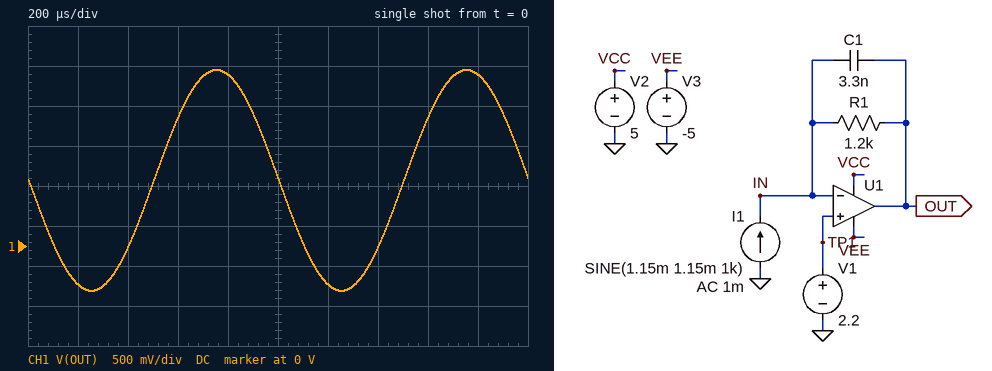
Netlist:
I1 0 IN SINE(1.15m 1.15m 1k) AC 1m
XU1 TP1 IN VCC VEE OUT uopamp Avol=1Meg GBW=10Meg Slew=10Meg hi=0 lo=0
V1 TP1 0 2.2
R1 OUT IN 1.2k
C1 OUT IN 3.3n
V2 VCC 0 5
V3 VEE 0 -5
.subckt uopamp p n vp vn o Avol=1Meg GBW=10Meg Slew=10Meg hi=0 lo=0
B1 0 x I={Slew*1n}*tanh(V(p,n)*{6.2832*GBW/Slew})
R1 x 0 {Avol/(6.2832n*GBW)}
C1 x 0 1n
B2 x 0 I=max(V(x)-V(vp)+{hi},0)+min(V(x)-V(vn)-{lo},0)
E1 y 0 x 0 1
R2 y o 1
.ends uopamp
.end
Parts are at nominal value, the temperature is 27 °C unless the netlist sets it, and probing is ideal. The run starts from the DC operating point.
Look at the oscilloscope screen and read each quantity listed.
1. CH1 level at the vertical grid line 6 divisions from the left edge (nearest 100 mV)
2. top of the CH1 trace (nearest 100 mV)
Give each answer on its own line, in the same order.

-500 mV
2.2 V
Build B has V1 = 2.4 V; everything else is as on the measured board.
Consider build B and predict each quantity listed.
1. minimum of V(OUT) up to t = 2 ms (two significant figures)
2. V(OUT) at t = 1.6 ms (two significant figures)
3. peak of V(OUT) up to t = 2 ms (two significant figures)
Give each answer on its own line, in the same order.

-360 mV
1.8 V
2.4 V
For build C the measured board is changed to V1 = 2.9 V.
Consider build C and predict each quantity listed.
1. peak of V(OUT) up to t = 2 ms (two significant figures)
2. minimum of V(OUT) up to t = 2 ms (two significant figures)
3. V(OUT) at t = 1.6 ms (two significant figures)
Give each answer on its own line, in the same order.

2.9 V
140 mV
2.3 V
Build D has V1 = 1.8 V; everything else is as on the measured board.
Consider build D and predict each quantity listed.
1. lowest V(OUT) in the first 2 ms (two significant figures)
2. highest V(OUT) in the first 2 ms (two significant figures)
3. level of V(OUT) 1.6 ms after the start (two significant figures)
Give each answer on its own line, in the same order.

-960 mV
1.8 V
1.2 V
